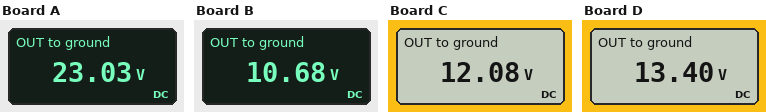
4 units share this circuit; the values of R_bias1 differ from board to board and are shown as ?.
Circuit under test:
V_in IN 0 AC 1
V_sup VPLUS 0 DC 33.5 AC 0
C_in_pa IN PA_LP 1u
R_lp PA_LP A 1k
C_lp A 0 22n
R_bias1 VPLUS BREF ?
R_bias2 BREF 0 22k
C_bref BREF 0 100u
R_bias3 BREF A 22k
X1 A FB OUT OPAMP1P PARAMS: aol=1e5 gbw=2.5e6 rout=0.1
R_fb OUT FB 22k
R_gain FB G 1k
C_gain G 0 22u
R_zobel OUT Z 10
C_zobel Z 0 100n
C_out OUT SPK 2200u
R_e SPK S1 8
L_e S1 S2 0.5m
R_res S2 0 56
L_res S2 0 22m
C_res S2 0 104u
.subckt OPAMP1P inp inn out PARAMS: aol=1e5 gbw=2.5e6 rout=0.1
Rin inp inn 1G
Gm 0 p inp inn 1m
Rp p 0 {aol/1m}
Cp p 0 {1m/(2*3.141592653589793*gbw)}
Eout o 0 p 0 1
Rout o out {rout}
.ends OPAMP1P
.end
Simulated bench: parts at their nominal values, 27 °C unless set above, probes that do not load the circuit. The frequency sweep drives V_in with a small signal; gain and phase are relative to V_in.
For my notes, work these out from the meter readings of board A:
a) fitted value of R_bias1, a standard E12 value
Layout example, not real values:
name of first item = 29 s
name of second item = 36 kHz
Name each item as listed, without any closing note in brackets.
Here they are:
fitted value of R_bias1, a standard E12 value = 10 kΩ
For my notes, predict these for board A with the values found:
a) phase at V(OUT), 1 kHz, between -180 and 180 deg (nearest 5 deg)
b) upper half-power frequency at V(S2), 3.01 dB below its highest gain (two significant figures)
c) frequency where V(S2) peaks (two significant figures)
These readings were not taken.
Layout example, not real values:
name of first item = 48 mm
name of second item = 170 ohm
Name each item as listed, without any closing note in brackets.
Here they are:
phase at V(OUT), 1 kHz, between -180 and 180 deg = -5 deg
upper half-power frequency at V(S2), 3.01 dB below its highest gain = 270 Hz
frequency where V(S2) peaks = 100 Hz
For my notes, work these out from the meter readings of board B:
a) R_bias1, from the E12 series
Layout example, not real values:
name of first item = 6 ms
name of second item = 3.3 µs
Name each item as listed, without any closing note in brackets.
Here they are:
R_bias1, from the E12 series = 47 kΩ
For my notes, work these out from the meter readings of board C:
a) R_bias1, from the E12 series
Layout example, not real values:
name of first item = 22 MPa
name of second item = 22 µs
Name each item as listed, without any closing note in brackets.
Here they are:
R_bias1, from the E12 series = 39 kΩ
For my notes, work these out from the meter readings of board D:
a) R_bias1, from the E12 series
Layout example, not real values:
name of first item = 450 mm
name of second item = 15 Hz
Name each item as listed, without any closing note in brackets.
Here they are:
R_bias1, from the E12 series = 33 kΩ
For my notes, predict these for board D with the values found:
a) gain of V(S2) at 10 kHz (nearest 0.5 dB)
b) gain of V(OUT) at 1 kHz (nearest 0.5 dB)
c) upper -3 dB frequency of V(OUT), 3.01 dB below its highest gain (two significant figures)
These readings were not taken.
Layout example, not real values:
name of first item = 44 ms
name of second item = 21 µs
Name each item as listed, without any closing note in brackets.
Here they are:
gain of V(S2) at 10 kHz = -24.0 dB
gain of V(OUT) at 1 kHz = 26.5 dB
upper -3 dB frequency of V(OUT), 3.01 dB below its highest gain = 7.7 kHz
